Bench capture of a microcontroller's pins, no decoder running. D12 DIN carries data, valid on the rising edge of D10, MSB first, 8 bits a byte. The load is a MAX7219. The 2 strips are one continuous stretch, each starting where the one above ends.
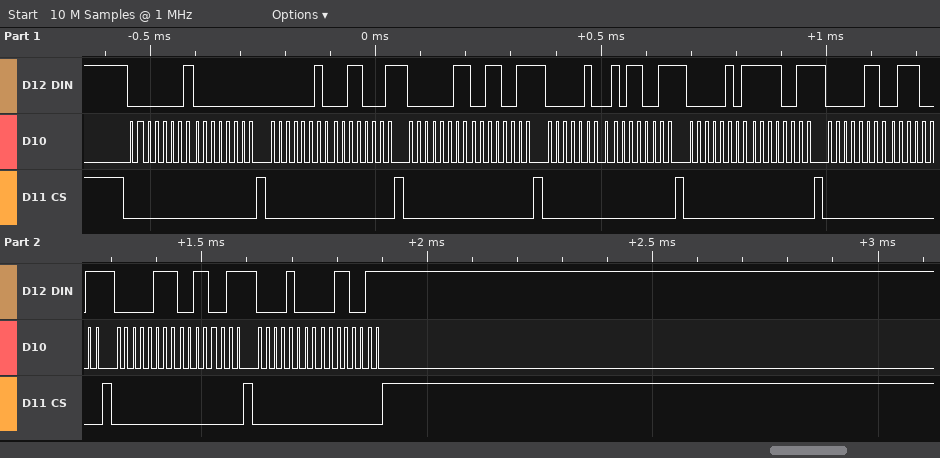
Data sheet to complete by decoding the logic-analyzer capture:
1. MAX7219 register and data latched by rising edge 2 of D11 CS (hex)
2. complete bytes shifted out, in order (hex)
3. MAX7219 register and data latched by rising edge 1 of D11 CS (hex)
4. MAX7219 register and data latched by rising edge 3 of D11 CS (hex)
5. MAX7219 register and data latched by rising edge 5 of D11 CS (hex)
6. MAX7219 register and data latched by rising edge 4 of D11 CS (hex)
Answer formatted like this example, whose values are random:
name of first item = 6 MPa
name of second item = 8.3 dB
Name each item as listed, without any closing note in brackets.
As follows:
MAX7219 register and data latched by rising edge 2 of D11 CS = register 0x2, data 0x31
complete bytes shifted out, in order = 01 00 02 31 03 33 04 B3 05 F3 06 73 07 33 08 33
MAX7219 register and data latched by rising edge 1 of D11 CS = register 0x1, data 0x00
MAX7219 register and data latched by rising edge 3 of D11 CS = register 0x3, data 0x33
MAX7219 register and data latched by rising edge 5 of D11 CS = register 0x5, data 0xF3
MAX7219 register and data latched by rising edge 4 of D11 CS = register 0x4, data 0xB3
